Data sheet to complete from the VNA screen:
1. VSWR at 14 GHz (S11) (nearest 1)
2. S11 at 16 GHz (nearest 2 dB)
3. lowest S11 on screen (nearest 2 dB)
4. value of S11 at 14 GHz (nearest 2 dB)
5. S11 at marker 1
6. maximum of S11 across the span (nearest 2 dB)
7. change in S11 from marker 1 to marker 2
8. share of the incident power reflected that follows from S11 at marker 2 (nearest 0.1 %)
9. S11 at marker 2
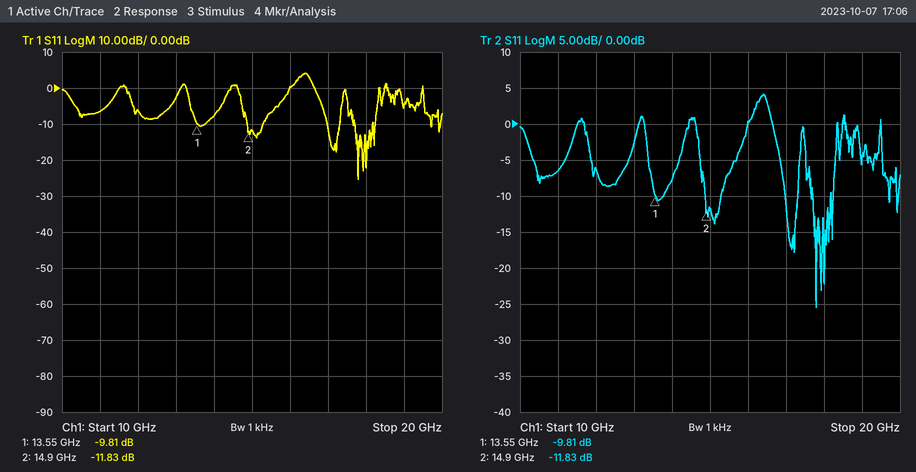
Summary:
2
0 dB
-26 dB
-8 dB
-9.81 dB
4 dB
-2.02 dB
6.6 %
-11.83 dB
